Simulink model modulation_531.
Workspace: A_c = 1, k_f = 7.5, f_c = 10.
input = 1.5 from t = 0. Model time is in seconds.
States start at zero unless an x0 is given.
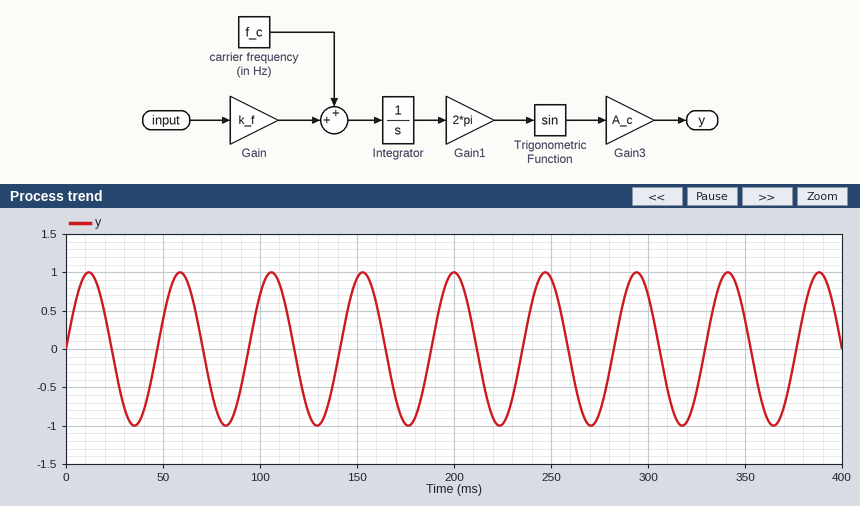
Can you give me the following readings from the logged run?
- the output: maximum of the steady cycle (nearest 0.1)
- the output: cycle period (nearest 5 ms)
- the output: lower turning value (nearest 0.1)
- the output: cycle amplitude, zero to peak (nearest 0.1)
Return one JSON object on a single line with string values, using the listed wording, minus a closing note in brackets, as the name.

{"the output: maximum of the steady cycle": "1.0", "the output: cycle period": "45 ms", "the output: lower turning value": "-1.0", "the output: cycle amplitude, zero to peak": "1.0"}
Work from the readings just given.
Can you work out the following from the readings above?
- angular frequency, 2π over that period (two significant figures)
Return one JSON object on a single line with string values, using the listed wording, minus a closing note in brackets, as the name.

{"angular frequency, 2π over that period": "0.14 rad/ms"}
